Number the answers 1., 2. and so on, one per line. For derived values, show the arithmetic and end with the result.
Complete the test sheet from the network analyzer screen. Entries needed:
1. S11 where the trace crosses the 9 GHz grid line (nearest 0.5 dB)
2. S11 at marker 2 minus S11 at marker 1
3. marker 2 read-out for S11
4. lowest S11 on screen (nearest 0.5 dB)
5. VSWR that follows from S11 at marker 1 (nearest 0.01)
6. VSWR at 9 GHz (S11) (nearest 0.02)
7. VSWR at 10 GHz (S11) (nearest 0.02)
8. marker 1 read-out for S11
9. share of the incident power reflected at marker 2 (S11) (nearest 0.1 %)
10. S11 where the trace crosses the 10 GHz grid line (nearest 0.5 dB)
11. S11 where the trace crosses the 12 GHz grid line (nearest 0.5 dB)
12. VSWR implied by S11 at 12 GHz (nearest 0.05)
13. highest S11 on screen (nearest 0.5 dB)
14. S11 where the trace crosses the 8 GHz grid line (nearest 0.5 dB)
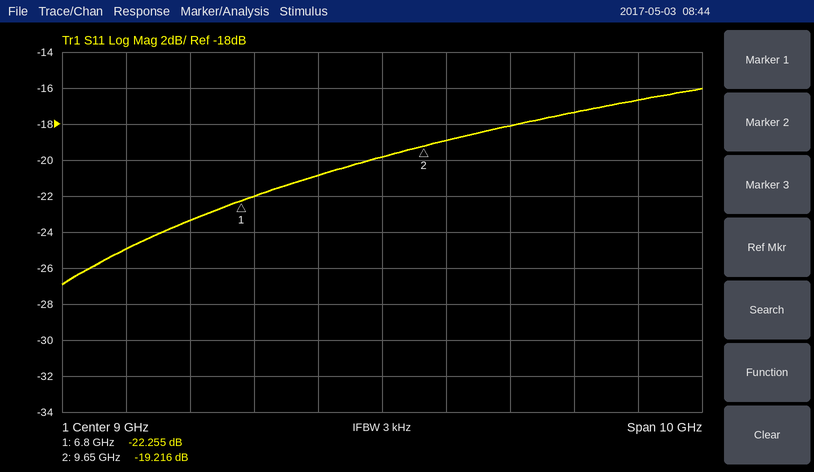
1. -20.0 dB
2. -19.216 − (-22.255) = 3.039 dB
3. -19.216 dB
4. -27.0 dB
5. (1 + 0.0771)/(1 − 0.0771) ≈ 1.17
6. |Γ| = 10^(-20/20) = 0.1000; VSWR = (1 + 0.1000)/(1 − 0.1000) ≈ 1.22
7. |Γ| = 10^(-19/20) = 0.1122; VSWR = (1 + 0.1122)/(1 − 0.1122) ≈ 1.25, so 1.26 to the nearest 0.02
8. -22.255 dB
9. 10^(-19.216/10) ≈ 1.2 %
10. -19.0 dB
11. -17.5 dB
12. |Γ| = 10^(-17.5/20) = 0.1334; VSWR = (1 + 0.1334)/(1 − 0.1334) ≈ 1.31, so 1.30 to the nearest 0.05
13. -16.0 dB
14. -21.0 dB
